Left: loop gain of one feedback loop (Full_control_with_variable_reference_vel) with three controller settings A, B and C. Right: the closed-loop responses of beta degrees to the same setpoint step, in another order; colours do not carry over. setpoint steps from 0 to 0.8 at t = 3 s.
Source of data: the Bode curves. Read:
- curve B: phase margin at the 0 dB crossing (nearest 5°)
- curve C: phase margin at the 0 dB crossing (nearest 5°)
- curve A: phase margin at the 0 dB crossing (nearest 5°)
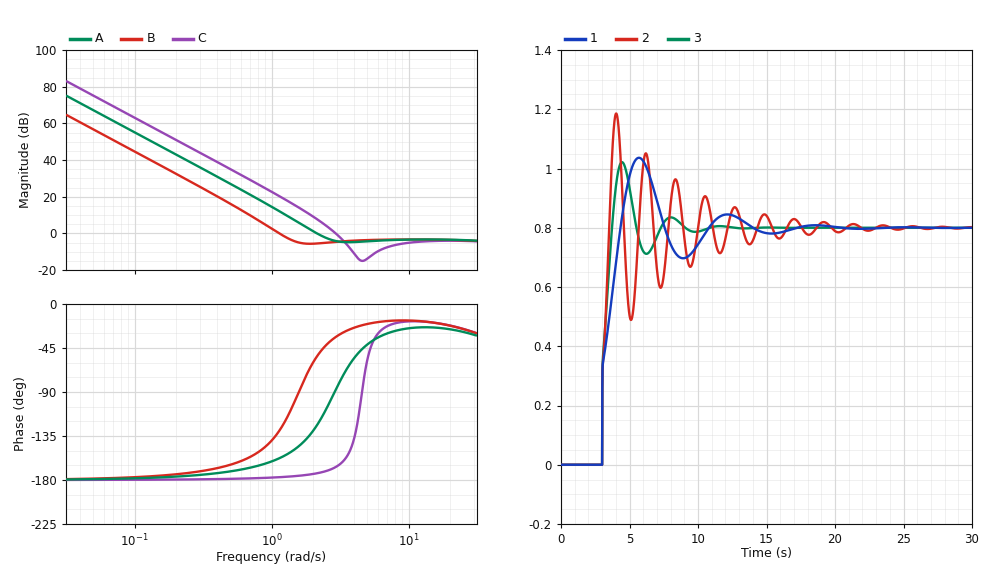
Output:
50°
15°
55°
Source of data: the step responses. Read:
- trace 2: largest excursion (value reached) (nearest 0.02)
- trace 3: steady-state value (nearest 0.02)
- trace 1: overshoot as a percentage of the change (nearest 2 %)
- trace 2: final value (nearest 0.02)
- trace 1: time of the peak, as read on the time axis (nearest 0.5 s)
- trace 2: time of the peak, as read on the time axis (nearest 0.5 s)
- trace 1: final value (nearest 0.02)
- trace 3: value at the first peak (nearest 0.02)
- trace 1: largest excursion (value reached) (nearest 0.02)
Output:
1.18
0.80
30 %
0.80
5.5 s
4.0 s
0.80
1.02
1.04
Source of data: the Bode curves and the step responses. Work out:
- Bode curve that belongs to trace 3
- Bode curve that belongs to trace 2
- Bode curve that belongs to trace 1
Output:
A
C
B
